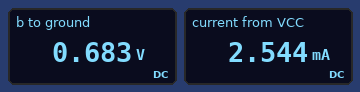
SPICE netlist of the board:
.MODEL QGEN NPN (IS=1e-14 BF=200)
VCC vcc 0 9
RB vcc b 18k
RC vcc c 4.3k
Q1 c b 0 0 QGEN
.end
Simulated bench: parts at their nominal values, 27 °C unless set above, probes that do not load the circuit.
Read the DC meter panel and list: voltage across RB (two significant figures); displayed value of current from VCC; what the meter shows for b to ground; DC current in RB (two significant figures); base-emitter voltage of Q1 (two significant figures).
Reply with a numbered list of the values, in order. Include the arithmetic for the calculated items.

1. 9 V - 683 mV = 8.3 V
2. 2.544 mA
3. 0.683 V
4. (9 V - 683 mV) / 18 kΩ = 460 µA
5. 683 mV = 680 mV
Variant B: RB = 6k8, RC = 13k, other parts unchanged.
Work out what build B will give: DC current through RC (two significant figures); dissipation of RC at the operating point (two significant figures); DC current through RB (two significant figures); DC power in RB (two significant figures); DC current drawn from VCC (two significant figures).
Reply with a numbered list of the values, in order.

1. 690 µA
2. 6.2 mW
3. 1.2 mA
4. 10 mW
5. 1.9 mA
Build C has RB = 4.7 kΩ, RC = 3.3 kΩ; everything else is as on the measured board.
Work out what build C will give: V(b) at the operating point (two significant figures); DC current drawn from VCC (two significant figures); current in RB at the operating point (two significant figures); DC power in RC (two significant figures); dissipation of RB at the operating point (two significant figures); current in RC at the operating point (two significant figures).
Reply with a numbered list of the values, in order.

1. 700 mV
2. 4.5 mA
3. 1.8 mA
4. 24 mW
5. 15 mW
6. 2.7 mA
